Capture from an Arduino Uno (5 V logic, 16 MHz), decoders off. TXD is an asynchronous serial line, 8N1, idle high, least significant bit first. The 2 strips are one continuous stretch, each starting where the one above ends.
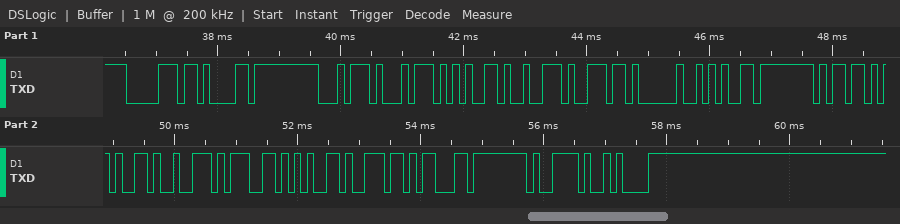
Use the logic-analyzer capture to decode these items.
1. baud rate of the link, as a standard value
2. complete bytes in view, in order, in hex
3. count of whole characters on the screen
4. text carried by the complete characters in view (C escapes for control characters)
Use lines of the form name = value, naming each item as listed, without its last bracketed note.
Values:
baud rate of the link, as a standard value = 9600 baud
complete bytes in view, in order, in hex = 70 61 74 74 65 72 6E 20 65 6D 65 72 67 65 6E 63 79 0A
count of whole characters on the screen = 18
text carried by the complete characters in view = "pattern emergency\n"
